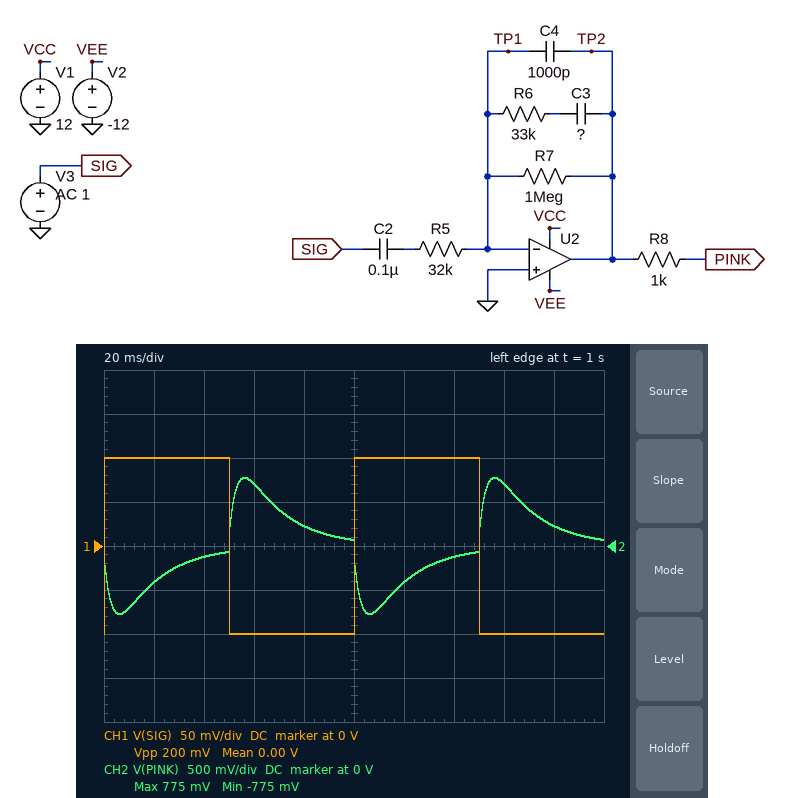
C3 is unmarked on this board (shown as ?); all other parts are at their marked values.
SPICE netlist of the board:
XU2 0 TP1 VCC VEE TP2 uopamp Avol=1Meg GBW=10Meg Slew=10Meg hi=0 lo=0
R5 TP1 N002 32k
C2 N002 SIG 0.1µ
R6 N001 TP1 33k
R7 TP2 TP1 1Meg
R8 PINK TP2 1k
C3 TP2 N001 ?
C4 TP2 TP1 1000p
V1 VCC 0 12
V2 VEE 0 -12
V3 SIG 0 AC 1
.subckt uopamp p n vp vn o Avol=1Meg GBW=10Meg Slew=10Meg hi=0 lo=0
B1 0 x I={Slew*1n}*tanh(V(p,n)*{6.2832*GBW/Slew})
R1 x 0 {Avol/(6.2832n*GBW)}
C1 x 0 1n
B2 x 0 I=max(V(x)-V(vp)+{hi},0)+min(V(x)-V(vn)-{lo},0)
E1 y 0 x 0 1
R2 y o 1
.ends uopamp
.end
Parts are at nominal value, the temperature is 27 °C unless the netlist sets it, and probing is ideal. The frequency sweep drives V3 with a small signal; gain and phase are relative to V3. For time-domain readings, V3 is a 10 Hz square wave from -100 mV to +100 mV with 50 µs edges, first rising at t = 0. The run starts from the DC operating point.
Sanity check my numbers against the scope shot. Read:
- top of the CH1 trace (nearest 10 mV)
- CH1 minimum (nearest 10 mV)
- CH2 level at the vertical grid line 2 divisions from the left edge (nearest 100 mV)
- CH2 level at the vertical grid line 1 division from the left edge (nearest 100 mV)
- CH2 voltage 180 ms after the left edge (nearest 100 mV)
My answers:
100 mV
-100 mV
-100 mV
-400 mV
200 mV
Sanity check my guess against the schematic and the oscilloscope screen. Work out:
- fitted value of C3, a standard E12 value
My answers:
15 nF
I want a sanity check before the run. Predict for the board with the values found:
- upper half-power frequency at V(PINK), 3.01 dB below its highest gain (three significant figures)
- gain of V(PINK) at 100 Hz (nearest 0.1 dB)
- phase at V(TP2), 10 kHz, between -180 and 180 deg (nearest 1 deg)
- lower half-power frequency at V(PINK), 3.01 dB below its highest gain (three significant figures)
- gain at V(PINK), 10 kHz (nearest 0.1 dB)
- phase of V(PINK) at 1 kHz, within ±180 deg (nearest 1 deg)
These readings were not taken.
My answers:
68.8 Hz
9.0 dB
116 deg
7.24 Hz
-7.1 dB
155 deg
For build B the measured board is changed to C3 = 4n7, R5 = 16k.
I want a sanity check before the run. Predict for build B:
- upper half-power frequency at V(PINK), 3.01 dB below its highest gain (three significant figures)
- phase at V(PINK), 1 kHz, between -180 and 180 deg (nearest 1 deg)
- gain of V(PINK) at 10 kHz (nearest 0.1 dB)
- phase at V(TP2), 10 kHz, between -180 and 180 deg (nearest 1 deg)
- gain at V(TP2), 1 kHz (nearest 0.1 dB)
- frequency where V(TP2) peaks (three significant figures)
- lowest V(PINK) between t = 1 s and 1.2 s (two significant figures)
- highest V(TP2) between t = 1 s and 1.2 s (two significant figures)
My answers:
147 Hz
132 deg
-1.3 dB
116 deg
7.4 dB
52.3 Hz
-2.1 V
2.1 V
